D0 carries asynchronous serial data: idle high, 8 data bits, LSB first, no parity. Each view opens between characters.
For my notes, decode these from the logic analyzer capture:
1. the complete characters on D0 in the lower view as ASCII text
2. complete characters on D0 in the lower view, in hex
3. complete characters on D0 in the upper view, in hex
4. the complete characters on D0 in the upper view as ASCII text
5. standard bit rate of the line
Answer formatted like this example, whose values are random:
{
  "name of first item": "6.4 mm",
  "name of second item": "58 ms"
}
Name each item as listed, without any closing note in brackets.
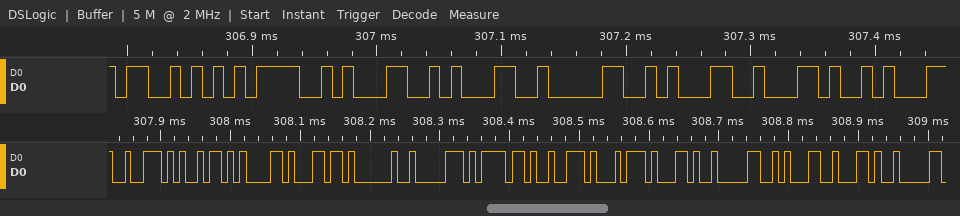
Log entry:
{
  "the complete characters on D0 in the lower view as ASCII text": "\"rial port,01,\"",
  "complete characters on D0 in the lower view, in hex": "72, 69, 61, 6C, 20, 70, 6F, 72, 74, 2C, 30, 31, 2C",
  "complete characters on D0 in the upper view, in hex": "53, 3D, 31, 31, 30, 31, 2C",
  "the complete characters on D0 in the upper view as ASCII text": "\"S=1101,\"",
  "standard bit rate of the line": "115200 baud"
}
